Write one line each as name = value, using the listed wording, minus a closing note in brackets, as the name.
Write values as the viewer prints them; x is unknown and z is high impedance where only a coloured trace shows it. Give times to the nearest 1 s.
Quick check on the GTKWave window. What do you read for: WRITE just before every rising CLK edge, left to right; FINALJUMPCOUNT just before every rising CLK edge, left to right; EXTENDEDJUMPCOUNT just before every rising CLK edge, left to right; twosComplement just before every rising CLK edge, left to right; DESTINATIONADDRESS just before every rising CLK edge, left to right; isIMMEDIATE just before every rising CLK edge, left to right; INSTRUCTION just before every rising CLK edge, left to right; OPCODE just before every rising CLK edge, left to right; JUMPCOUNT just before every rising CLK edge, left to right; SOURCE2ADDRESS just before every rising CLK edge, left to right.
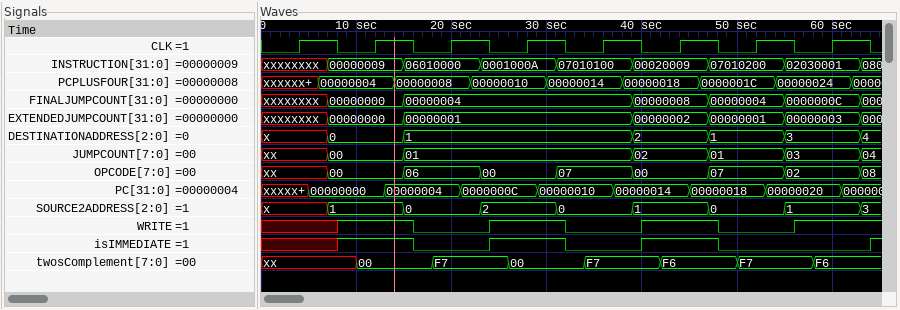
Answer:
WRITE just before every rising CLK edge, left to right = x 1 0 1 0 1 0 1
FINALJUMPCOUNT just before every rising CLK edge, left to right = xxxxxxxx, 00000000, 00000004, 00000004, 00000004, 00000008, 00000004, 0000000C
EXTENDEDJUMPCOUNT just before every rising CLK edge, left to right = xxxxxxxx, 00000000, 00000001, 00000001, 00000001, 00000002, 00000001, 00000003
twosComplement just before every rising CLK edge, left to right = xx, 00, F7, 00, F7, F6, F7, F6
DESTINATIONADDRESS just before every rising CLK edge, left to right = x, 0, 1, 1, 1, 2, 1, 3
isIMMEDIATE just before every rising CLK edge, left to right = x 1 0 1 0 1 0 0
INSTRUCTION just before every rising CLK edge, left to right = xxxxxxxx, 00000009, 06010000, 0001000A, 07010100, 00020009, 07010200, 02030001
OPCODE just before every rising CLK edge, left to right = xx, 00, 06, 00, 07, 00, 07, 02
JUMPCOUNT just before every rising CLK edge, left to right = xx, 00, 01, 01, 01, 02, 01, 03
SOURCE2ADDRESS just before every rising CLK edge, left to right = x, 1, 0, 2, 0, 1, 0, 1
